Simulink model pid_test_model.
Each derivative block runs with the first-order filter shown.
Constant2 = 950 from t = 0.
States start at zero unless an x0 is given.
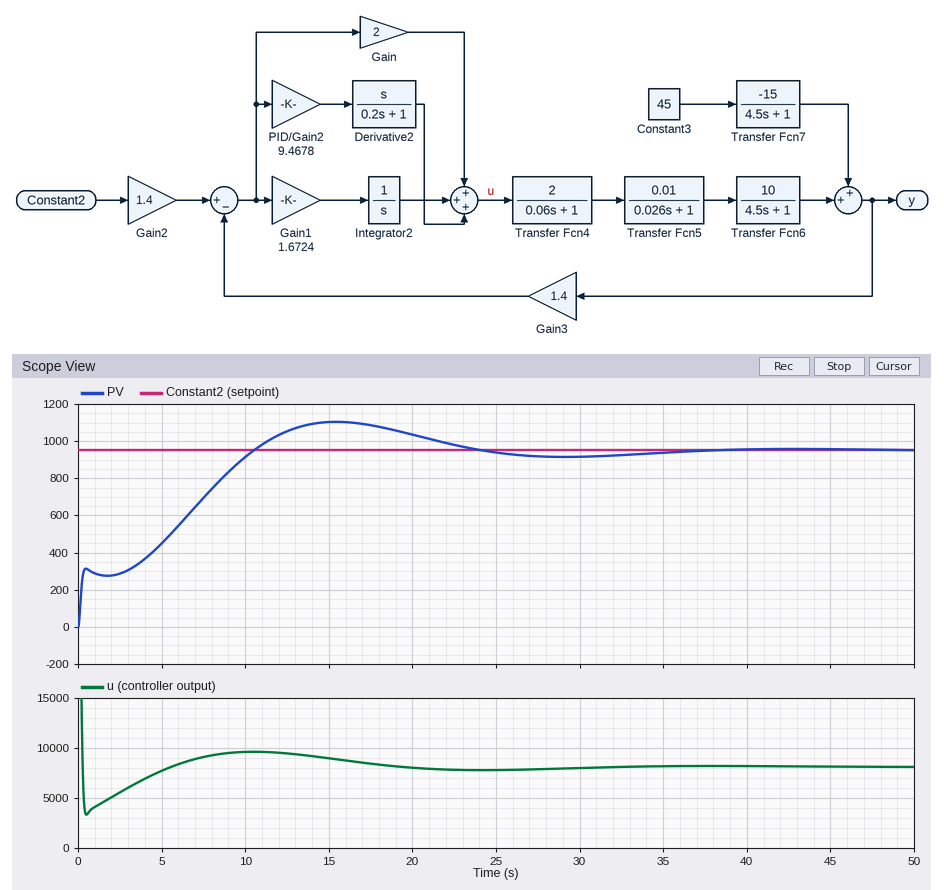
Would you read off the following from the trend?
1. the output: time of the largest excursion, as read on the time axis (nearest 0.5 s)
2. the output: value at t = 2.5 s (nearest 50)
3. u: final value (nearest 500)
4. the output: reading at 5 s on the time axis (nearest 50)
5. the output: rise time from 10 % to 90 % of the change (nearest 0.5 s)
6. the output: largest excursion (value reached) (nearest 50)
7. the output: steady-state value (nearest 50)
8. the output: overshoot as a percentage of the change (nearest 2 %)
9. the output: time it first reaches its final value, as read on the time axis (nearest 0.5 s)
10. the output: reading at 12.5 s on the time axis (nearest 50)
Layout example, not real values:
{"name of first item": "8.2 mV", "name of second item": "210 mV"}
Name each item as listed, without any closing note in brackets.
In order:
{"the output: time of the largest excursion, as read on the time axis": "15.5 s", "the output: value at t = 2.5 s": "300", "u: final value": "8000", "the output: reading at 5 s on the time axis": "450", "the output: rise time from 10 % to 90 % of the change": "9.0 s", "the output: largest excursion (value reached)": "1100", "the output: steady-state value": "950", "the output: overshoot as a percentage of the change": "16 %", "the output: time it first reaches its final value, as read on the time axis": "10.5 s", "the output: reading at 12.5 s on the time axis": "1050"}
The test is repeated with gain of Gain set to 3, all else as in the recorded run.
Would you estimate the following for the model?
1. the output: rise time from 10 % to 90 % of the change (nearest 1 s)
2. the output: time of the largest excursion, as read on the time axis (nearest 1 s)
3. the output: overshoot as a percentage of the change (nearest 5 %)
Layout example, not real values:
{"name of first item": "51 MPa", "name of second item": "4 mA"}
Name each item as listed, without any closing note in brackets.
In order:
{"the output: rise time from 10 % to 90 % of the change": "9 s", "the output: time of the largest excursion, as read on the time axis": "16 s", "the output: overshoot as a percentage of the change": "10 %"}
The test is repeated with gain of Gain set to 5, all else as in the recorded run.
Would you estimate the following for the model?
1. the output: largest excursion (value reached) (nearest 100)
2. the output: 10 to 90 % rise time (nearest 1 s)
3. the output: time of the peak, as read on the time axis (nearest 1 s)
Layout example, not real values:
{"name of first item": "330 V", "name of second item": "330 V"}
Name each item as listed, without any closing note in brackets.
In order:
{"the output: largest excursion (value reached)": "1000", "the output: 10 to 90 % rise time": "9 s", "the output: time of the peak, as read on the time axis": "17 s"}
